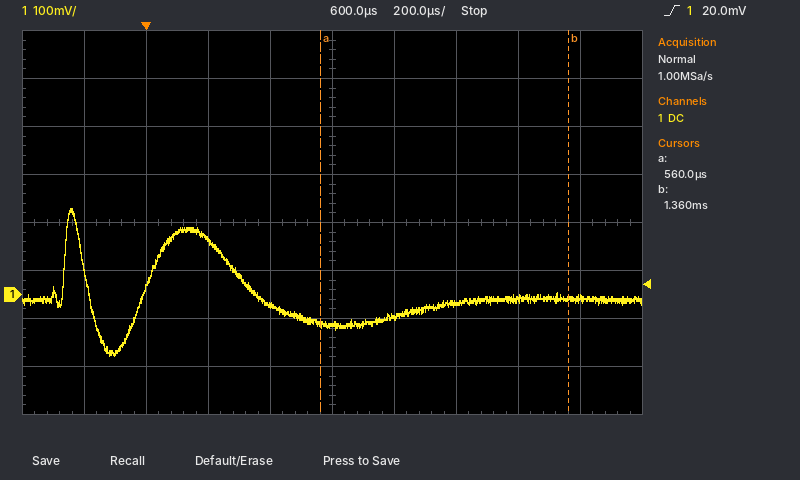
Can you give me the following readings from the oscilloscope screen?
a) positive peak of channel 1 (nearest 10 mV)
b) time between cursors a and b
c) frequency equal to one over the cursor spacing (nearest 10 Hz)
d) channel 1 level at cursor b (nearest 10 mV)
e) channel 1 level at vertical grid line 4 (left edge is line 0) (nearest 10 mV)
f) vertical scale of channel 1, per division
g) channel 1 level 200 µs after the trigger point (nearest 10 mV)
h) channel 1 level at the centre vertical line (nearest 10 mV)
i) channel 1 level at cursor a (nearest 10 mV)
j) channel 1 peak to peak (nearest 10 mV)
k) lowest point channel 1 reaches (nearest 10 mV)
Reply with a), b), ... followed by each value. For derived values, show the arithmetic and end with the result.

a) 180 mV
b) 1.36 ms − (560 µs) = 800 µs
c) 1 / 800 µs ≈ 1.25 kHz
d) -10 mV
e) -20 mV
f) 100 mV
g) 110 mV
h) -60 mV
i) -60 mV
j) 180 mV − (-130 mV) = 310 mV
k) -130 mV
